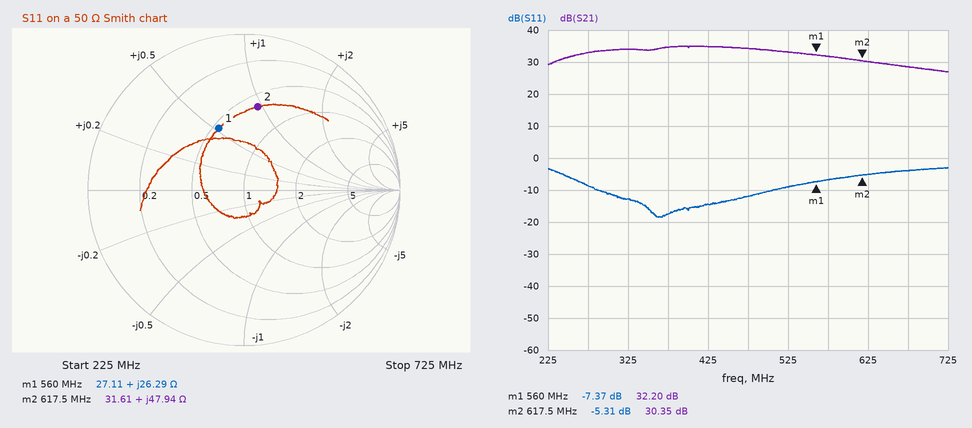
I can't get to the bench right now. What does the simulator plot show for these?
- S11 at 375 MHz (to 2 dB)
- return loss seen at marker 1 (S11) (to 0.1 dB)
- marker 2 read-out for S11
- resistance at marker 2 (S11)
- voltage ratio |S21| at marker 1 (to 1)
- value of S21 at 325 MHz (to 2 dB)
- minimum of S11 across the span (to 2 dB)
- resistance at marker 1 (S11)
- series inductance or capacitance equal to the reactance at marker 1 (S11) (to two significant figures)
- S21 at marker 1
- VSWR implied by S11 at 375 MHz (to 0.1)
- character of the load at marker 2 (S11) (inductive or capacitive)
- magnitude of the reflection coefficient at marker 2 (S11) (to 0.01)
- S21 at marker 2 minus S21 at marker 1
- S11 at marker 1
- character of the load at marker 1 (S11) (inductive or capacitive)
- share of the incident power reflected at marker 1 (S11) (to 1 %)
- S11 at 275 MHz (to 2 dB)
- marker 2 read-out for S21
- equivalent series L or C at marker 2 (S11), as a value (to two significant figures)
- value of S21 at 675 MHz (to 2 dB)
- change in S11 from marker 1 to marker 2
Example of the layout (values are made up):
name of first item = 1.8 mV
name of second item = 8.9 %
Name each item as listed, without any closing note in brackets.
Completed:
S11 at 375 MHz = -18 dB
return loss seen at marker 1 (S11) = 7.4 dB
marker 2 read-out for S11 = -5.31 dB
resistance at marker 2 = 31.61 Ω
voltage ratio |S21| at marker 1 = 41
value of S21 at 325 MHz = 34 dB
minimum of S11 across the span = -18 dB
resistance at marker 1 = 27.11 Ω
series inductance or capacitance equal to the reactance at marker 1 (S11) = 7.5 nH
S21 at marker 1 = 32.20 dB
VSWR implied by S11 at 375 MHz = 1.3
character of the load at marker 2 (S11) = inductive
magnitude of the reflection coefficient at marker 2 (S11) = 0.54
S21 at marker 2 minus S21 at marker 1 = -1.85 dB
S11 at marker 1 = -7.37 dB
character of the load at marker 1 (S11) = inductive
share of the incident power reflected at marker 1 (S11) = 18 %
S11 at 275 MHz = -8 dB
marker 2 read-out for S21 = 30.35 dB
equivalent series L or C at marker 2 (S11), as a value = 12 nH
value of S21 at 675 MHz = 28 dB
change in S11 from marker 1 to marker 2 = 2.06 dB
